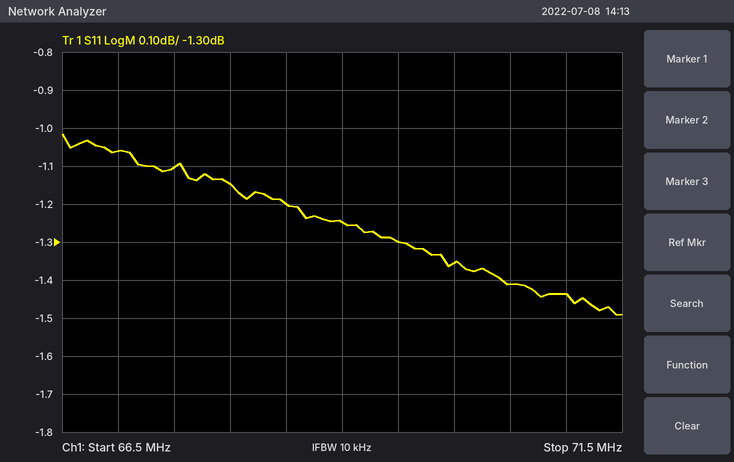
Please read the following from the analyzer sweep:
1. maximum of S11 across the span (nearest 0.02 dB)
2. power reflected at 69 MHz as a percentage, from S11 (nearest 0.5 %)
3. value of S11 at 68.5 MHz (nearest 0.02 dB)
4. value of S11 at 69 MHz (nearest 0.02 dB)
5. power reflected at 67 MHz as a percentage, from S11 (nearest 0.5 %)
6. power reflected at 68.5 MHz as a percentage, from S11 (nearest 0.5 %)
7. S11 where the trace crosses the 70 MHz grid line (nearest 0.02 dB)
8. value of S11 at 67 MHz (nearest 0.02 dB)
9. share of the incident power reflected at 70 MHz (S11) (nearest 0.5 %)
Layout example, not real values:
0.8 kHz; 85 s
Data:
-1.02 dB; 75.0 %; -1.20 dB; -1.24 dB; 78.5 %; 76.0 %; -1.36 dB; -1.06 dB; 73.0 %
